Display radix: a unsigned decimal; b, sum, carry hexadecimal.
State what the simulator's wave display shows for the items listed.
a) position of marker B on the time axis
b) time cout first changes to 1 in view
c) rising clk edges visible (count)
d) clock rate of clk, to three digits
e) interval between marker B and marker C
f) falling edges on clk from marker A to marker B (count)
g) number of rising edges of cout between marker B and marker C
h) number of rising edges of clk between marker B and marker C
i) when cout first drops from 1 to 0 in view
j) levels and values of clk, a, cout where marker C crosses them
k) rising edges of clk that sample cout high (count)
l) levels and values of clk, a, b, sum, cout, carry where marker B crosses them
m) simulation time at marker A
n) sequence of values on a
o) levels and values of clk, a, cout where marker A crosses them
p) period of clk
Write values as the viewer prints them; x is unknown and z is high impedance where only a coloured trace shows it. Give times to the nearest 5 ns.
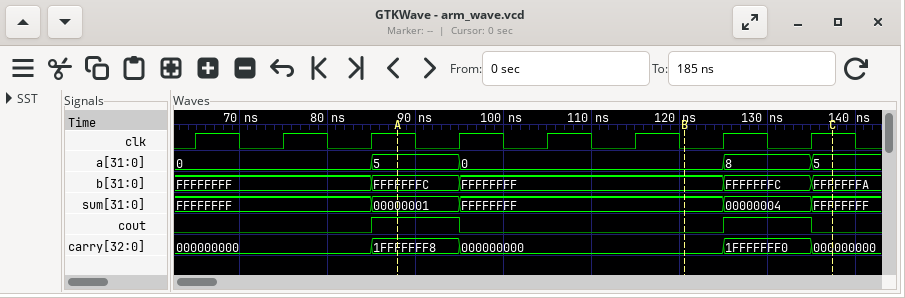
120 ns
85 ns
8
100 MHz
15 ns
4
1
2
95 ns
clk=1, a=5, cout=0
2
clk=0, a=0, b=FFFFFFFF, sum=FFFFFFFF, cout=0, carry=000000000
90 ns
0, 5, 0, 8, 5
clk=1, a=5, cout=1
10 ns
